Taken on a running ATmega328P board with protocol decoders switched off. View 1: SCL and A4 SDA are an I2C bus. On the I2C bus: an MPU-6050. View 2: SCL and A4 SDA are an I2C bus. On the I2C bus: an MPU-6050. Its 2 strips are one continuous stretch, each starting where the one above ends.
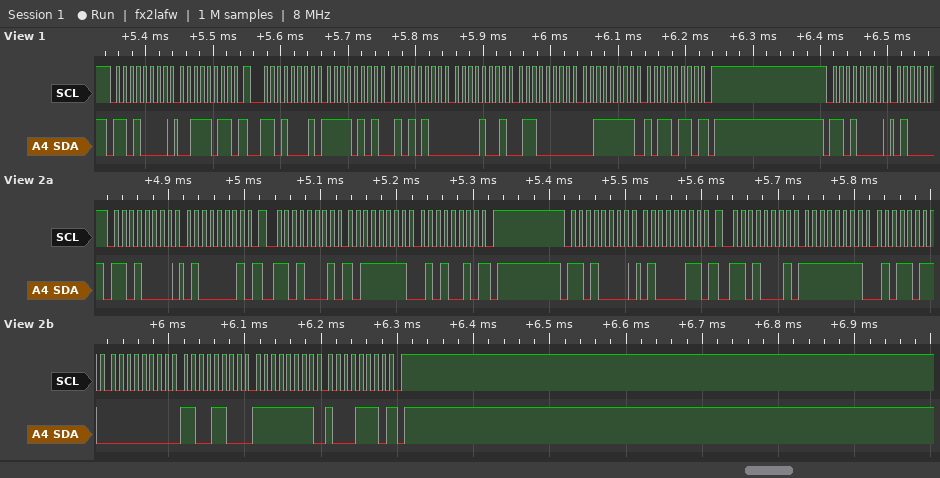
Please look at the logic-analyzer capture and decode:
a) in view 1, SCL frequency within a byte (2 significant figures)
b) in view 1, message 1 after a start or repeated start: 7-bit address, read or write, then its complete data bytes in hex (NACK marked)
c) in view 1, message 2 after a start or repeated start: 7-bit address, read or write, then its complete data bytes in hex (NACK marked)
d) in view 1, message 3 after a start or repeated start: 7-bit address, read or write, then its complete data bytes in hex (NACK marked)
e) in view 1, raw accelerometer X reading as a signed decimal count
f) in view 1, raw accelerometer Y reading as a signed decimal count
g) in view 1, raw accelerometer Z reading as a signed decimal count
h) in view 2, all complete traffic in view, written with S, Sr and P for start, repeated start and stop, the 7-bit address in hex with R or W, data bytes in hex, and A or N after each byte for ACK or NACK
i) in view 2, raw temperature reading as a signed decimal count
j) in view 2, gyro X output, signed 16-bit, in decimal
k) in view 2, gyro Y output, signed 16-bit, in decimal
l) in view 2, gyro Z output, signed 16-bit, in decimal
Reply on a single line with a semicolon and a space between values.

100 kHz; 0x68 write: 3B; 0x68 read: F5 54 09 60 3F B6 NACK; 0x68 write; -2732; 2400; 16310; S 68W A 41 A Sr 68R A BF A 52 N P S 68W A 43 A Sr 68R A FF A 5B A 00 A CC A FF A 8E N P; -16558; -165; 204; -114
